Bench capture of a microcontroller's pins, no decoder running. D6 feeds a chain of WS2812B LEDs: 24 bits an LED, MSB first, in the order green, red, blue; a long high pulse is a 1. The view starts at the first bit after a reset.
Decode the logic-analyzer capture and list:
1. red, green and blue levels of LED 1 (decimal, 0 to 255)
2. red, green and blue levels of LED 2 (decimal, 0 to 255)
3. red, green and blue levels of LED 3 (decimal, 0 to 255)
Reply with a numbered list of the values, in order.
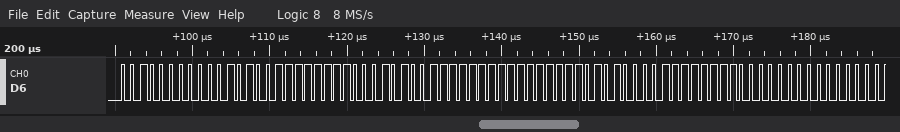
1. 20, 32, 255
2. 255, 20, 255
3. 255, 80, 0
